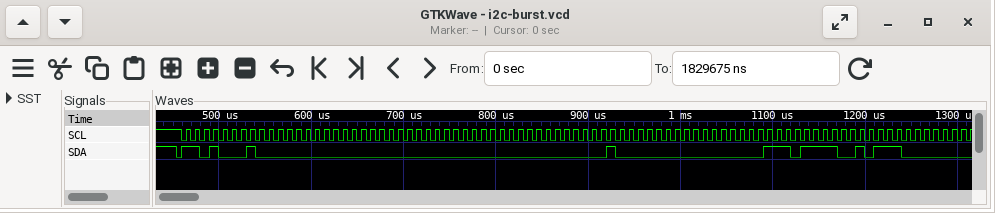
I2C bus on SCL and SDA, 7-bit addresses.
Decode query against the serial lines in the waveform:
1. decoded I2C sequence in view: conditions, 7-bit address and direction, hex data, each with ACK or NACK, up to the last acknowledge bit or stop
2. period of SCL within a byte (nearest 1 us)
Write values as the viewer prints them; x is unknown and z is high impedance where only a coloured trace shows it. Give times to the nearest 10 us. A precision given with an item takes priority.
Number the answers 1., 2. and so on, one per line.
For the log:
1. start, address 68 read ACK, 00 ACK, 00 ACK, 00 ACK, 00 ACK, 40 ACK, 00 ACK, EF ACK, 5C ACK
2. 10 us
